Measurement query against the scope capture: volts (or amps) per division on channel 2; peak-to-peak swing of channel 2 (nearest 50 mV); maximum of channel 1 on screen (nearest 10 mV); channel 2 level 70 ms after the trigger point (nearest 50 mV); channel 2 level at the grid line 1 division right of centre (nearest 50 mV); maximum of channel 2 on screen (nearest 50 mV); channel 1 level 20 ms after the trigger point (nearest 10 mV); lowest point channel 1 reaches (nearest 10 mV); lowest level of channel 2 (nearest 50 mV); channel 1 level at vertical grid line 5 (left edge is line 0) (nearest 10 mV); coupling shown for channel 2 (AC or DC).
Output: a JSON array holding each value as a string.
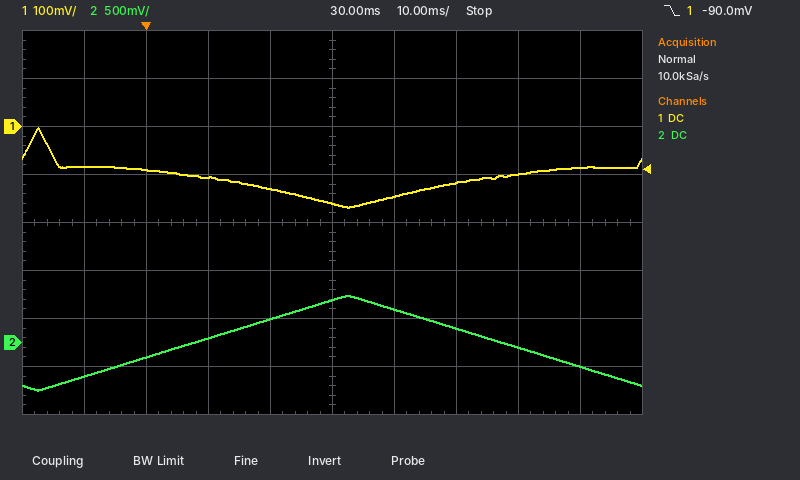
["500 mV", "1.00 V", "0 mV", "-250 mV", "350 mV", "500 mV", "-130 mV", "-170 mV", "-500 mV", "-160 mV", "DC"]
